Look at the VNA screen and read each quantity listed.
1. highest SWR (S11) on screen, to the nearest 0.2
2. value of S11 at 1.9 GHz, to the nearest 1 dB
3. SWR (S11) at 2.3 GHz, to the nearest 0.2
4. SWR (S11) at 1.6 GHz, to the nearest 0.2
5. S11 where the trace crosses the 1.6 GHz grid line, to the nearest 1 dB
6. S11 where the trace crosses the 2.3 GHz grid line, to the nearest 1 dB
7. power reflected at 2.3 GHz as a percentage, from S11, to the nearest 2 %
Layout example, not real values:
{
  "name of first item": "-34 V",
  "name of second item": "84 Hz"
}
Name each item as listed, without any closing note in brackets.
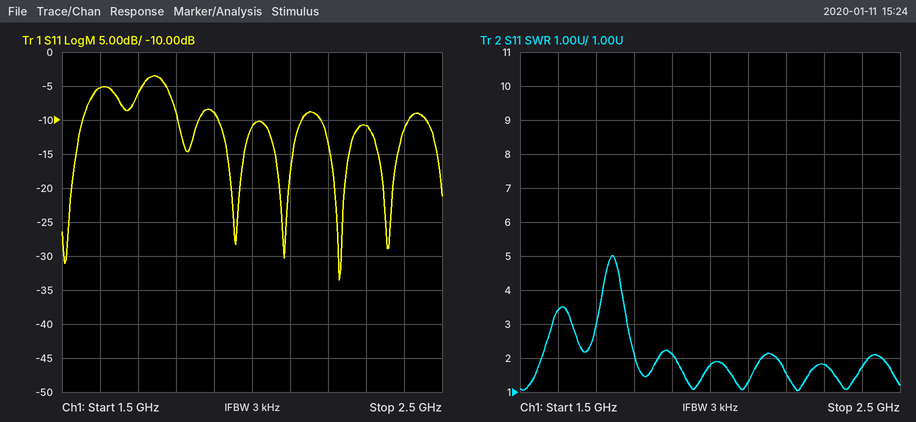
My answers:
{
  "highest SWR (S11) on screen, to the nearest 0.2": "5.0",
  "value of S11 at 1.9 GHz, to the nearest 1 dB": "-9 dB",
  "SWR (S11) at 2.3 GHz, to the nearest 0.2": "1.8",
  "SWR (S11) at 1.6 GHz, to the nearest 0.2": "3.4",
  "S11 where the trace crosses the 1.6 GHz grid line, to the nearest 1 dB": "-5 dB",
  "S11 where the trace crosses the 2.3 GHz grid line, to the nearest 1 dB": "-11 dB",
  "power reflected at 2.3 GHz as a percentage, from S11, to the nearest 2 %": "8 %"
}
